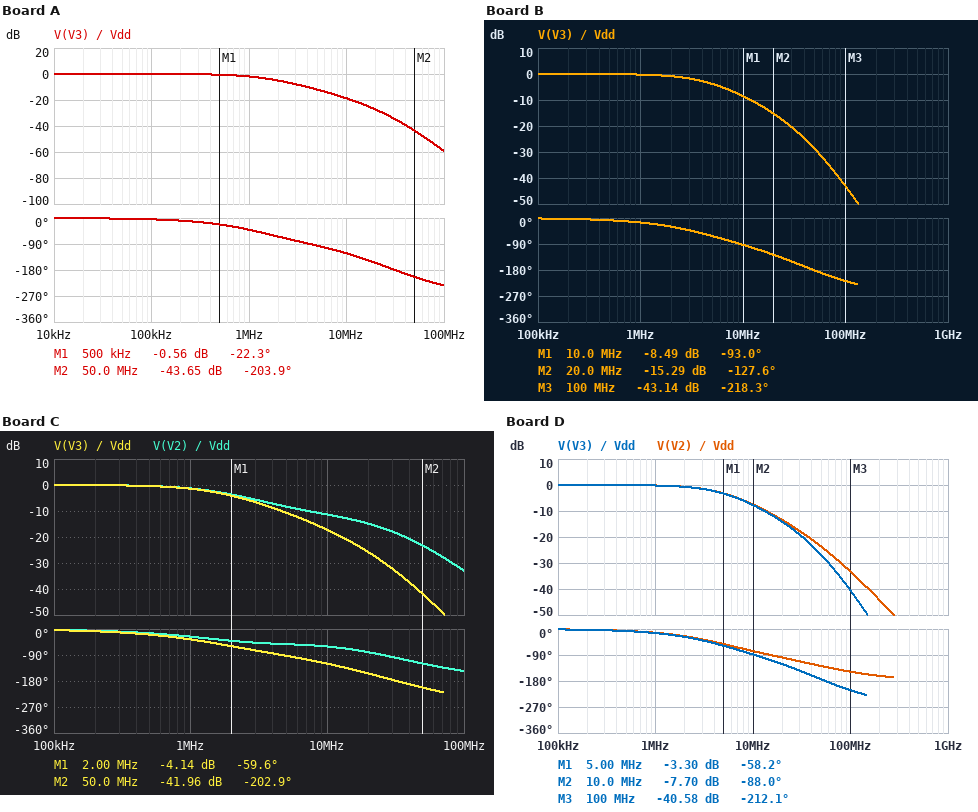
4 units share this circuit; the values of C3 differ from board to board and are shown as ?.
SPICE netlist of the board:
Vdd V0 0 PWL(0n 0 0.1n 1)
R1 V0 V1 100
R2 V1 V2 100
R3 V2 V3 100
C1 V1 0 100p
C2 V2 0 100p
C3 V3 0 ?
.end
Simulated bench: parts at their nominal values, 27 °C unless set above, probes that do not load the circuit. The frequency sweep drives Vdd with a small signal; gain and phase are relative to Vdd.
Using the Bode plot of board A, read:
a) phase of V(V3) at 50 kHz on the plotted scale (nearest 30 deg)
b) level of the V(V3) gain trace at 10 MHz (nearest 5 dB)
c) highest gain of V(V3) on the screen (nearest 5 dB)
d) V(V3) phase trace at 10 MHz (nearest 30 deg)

0 deg
-20 dB
0 dB
-120 deg
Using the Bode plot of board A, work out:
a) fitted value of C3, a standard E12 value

330 pF
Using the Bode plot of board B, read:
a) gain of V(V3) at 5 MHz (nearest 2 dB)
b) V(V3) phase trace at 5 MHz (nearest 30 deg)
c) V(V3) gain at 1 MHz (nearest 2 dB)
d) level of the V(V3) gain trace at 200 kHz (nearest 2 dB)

-4 dB
-60 deg
0 dB
0 dB
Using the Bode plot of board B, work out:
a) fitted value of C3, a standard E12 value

47 pF
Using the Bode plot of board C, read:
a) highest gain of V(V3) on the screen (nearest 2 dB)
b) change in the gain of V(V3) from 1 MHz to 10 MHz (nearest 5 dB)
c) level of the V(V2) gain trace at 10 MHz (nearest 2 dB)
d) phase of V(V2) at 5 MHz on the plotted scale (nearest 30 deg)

0 dB
-15 dB
-12 dB
-60 deg
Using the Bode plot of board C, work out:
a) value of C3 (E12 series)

270 pF
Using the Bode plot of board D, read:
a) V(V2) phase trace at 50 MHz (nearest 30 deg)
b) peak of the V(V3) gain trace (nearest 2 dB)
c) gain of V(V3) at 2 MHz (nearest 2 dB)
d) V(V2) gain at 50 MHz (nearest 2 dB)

-120 deg
0 dB
0 dB
-24 dB
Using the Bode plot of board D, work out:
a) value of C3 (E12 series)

33 pF
